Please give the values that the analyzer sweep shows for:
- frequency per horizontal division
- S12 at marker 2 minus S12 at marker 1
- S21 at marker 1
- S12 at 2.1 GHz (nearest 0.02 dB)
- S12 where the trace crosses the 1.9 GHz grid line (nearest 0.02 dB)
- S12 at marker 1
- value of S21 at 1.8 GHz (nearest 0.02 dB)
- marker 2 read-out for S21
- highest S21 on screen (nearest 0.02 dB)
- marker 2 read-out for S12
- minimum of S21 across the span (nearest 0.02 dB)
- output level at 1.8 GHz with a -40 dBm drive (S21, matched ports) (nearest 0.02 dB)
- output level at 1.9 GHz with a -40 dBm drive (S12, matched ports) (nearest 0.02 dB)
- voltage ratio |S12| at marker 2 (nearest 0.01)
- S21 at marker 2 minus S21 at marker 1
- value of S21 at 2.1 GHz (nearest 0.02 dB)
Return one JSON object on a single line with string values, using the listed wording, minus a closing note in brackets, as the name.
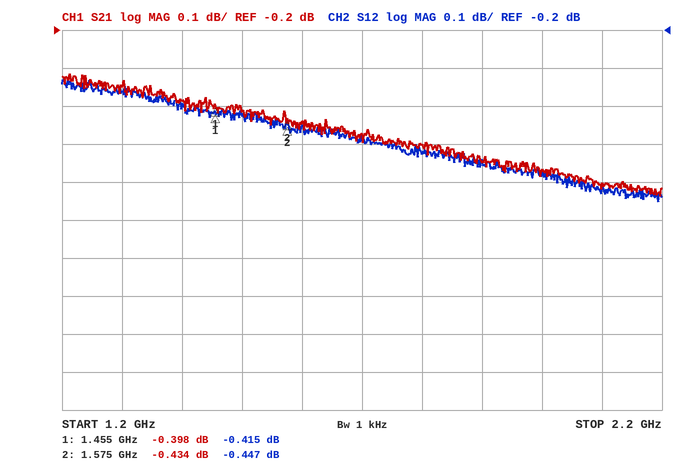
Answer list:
{"frequency per horizontal division": "100 MHz", "S12 at marker 2 minus S12 at marker 1": "-0.032 dB", "S21 at marker 1": "-0.398 dB", "S12 at 2.1 GHz": "-0.62 dB", "S12 where the trace crosses the 1.9 GHz grid line": "-0.54 dB", "S12 at marker 1": "-0.415 dB", "value of S21 at 1.8 GHz": "-0.50 dB", "marker 2 read-out for S21": "-0.434 dB", "highest S21 on screen": "-0.32 dB", "marker 2 read-out for S12": "-0.447 dB", "minimum of S21 across the span": "-0.64 dB", "output level at 1.8 GHz with a -40 dBm drive (S21, matched ports)": "-40.50 dBm", "output level at 1.9 GHz with a -40 dBm drive (S12, matched ports)": "-40.54 dBm", "voltage ratio |S12| at marker 2": "0.95", "S21 at marker 2 minus S21 at marker 1": "-0.036 dB", "value of S21 at 2.1 GHz": "-0.60 dB"}
